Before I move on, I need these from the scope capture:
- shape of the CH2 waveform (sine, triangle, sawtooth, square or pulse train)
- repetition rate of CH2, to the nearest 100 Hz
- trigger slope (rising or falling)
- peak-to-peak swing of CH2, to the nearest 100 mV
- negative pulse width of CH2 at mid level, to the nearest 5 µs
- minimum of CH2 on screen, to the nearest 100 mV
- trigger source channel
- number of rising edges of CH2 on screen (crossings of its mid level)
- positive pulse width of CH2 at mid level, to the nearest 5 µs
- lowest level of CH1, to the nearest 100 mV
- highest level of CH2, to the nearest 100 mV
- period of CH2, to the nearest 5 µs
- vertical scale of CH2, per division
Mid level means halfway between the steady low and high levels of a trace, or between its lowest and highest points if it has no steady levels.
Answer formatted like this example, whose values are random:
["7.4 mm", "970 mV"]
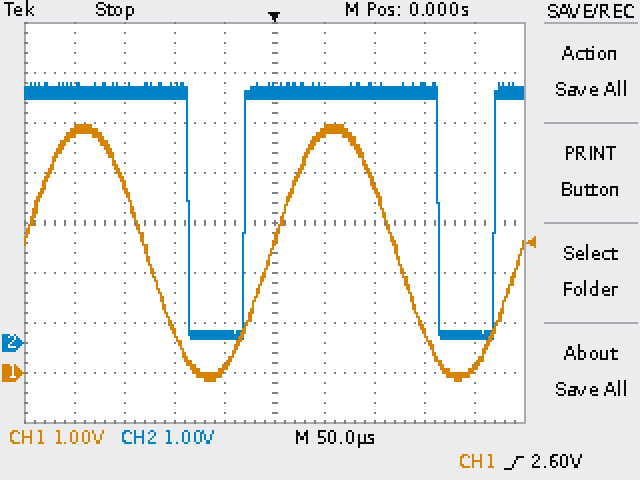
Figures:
["pulse train", "4.0 kHz", "rising", "5.1 V", "55 µs", "100 mV", "CH1", "2", "195 µs", "-200 mV", "5.2 V", "250 µs", "1 V"]
